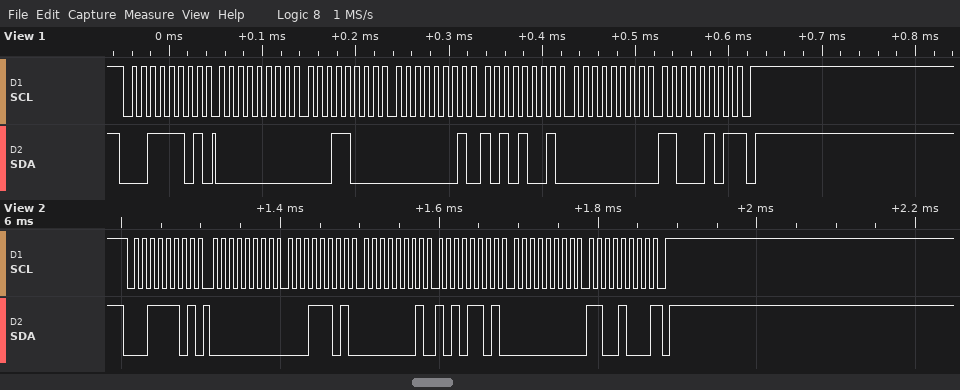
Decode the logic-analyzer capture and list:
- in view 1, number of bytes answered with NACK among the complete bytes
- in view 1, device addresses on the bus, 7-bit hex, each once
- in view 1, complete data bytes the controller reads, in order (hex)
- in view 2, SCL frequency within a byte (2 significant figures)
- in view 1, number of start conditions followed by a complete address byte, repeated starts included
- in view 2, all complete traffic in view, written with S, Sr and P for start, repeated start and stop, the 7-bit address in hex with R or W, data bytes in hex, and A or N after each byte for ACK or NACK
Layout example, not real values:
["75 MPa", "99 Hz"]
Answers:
["1", "0x1E", "00 18 01 A9 00 C5", "100 kHz", "1", "S 1ER A 00 A 1D A 01 A AD A 00 A C8 N P"]
